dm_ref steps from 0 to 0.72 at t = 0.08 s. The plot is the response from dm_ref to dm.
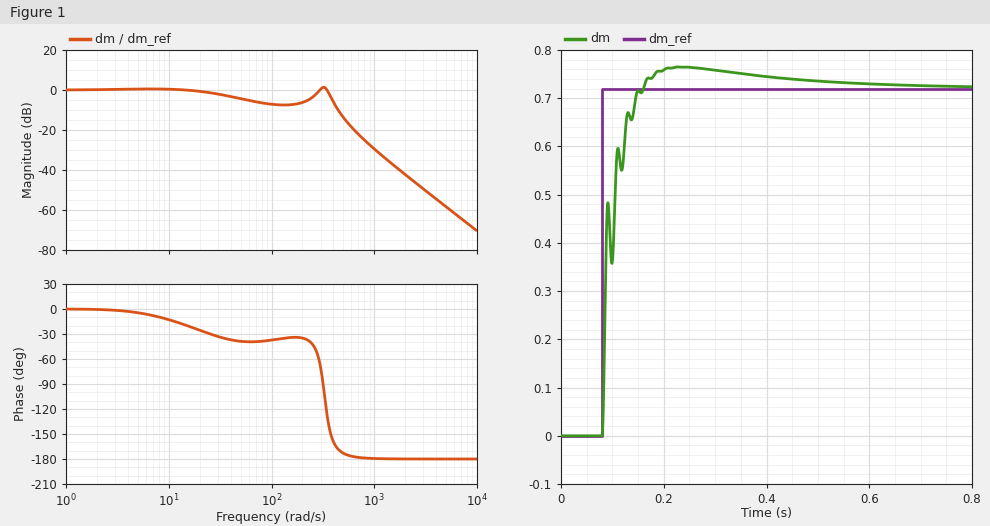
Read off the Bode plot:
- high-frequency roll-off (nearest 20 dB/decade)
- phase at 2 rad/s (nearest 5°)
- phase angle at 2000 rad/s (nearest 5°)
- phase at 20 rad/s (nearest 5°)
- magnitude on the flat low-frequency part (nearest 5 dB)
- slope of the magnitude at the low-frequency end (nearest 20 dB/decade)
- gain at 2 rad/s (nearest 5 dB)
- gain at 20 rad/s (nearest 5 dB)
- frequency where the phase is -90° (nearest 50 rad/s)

-40 dB/decade
0°
-180°
-25°
0 dB
0 dB/decade
0 dB
0 dB
300 rad/s
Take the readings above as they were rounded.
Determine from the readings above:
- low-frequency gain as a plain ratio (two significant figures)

1.0
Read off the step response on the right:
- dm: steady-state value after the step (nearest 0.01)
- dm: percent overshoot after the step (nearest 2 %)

0.72
6 %
